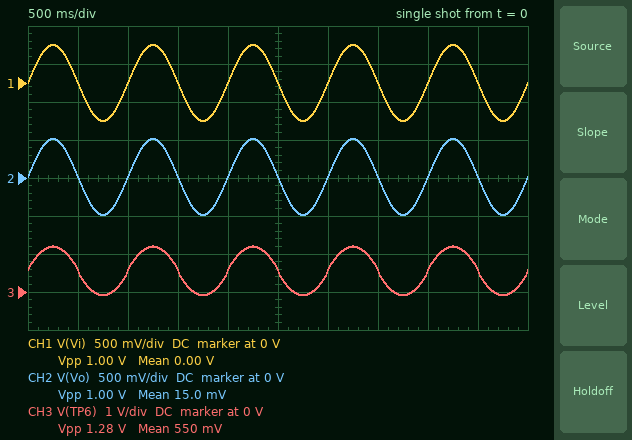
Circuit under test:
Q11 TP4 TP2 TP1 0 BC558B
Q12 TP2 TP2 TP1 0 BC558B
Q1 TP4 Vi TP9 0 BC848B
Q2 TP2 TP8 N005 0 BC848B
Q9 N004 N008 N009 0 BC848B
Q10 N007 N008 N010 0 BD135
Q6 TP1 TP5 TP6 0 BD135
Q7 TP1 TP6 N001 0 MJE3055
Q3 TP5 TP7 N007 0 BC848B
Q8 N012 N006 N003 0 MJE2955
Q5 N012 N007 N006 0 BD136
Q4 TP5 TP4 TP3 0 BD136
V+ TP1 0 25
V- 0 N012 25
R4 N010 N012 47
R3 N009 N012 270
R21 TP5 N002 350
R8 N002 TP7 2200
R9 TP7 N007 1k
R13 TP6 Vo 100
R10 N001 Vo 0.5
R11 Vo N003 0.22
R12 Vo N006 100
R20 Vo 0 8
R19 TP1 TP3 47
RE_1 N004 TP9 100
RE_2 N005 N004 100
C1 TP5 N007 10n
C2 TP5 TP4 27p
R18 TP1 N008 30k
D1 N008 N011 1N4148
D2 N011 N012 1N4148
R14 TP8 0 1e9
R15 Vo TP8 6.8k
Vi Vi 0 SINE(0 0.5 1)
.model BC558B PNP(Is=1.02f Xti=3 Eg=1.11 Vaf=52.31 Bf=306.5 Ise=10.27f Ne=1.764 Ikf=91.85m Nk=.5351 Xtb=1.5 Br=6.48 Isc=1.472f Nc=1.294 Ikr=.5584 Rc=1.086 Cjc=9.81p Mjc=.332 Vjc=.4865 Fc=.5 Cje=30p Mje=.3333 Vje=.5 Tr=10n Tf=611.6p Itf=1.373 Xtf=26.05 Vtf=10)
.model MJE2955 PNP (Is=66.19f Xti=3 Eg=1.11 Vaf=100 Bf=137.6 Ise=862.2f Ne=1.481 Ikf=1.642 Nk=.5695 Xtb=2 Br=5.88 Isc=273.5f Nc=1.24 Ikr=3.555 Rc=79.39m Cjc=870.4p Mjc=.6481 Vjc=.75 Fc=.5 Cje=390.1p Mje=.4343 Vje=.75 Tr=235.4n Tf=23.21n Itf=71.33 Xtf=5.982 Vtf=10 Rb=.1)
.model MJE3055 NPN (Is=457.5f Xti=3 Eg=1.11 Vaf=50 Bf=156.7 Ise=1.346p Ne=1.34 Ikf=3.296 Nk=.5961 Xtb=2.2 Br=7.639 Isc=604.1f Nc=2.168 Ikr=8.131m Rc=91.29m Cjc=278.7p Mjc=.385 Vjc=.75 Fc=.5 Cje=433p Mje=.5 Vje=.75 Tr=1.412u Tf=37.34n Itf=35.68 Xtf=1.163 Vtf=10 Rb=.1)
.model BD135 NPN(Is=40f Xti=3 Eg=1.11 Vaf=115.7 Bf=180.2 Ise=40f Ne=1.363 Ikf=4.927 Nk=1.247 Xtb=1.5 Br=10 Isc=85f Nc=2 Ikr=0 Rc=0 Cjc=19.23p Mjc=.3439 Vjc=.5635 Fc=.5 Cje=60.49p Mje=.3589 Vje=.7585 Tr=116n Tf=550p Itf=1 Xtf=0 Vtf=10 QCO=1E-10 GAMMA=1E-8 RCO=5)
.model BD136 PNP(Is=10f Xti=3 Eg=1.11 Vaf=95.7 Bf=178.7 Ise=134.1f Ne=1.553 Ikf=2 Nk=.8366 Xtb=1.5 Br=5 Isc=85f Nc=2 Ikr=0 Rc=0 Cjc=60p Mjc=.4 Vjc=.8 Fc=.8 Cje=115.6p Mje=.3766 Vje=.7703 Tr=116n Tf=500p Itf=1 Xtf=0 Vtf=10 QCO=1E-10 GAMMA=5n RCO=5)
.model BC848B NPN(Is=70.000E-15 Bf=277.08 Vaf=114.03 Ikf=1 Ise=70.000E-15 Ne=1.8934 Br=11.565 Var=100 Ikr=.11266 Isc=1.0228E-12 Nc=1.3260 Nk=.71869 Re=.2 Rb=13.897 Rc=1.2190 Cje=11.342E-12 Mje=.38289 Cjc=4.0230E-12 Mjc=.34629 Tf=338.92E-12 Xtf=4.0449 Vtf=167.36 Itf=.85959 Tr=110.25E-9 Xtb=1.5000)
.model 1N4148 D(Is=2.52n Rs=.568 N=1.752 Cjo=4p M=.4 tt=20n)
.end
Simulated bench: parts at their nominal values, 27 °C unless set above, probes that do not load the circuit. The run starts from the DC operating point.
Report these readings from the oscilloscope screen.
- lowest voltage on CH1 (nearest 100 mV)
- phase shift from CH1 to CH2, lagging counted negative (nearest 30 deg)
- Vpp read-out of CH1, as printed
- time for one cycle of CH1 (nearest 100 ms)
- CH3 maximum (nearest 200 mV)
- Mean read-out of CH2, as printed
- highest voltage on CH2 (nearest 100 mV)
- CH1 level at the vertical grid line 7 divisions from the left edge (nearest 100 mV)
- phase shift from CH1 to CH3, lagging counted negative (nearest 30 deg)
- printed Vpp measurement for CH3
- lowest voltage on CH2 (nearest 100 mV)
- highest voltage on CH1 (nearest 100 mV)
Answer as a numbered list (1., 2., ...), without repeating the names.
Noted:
1. -500 mV
2. 0 deg
3. 1.00 V
4. 1.0 s
5. 1.2 V
6. 15.0 mV
7. 500 mV
8. 0 V
9. 0 deg
10. 1.28 V
11. -500 mV
12. 500 mV
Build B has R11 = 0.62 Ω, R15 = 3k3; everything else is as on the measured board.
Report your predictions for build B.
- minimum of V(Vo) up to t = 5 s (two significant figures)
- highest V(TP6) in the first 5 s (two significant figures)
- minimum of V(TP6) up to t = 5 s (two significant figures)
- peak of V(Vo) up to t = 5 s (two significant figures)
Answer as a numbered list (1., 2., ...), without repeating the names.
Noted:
1. -500 mV
2. 1.2 V
3. -120 mV
4. 500 mV
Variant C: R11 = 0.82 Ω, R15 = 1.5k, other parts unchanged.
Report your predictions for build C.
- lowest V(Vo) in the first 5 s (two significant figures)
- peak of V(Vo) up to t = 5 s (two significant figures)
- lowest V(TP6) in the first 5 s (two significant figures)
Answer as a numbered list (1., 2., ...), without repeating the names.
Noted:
1. -500 mV
2. 500 mV
3. -140 mV
